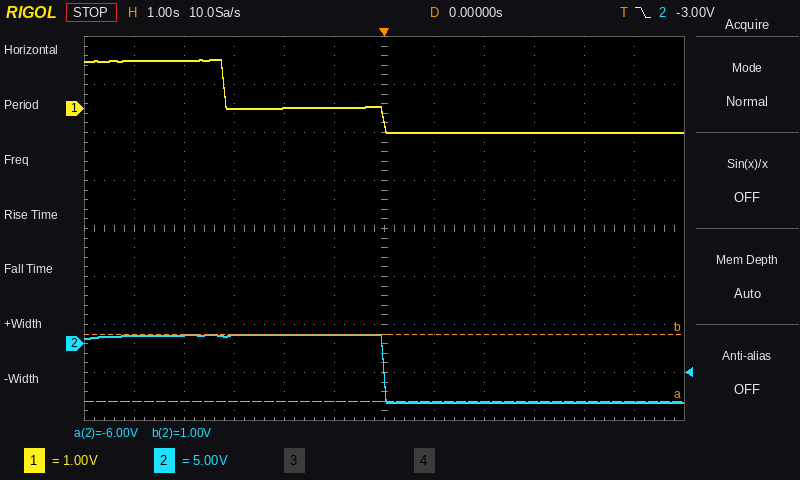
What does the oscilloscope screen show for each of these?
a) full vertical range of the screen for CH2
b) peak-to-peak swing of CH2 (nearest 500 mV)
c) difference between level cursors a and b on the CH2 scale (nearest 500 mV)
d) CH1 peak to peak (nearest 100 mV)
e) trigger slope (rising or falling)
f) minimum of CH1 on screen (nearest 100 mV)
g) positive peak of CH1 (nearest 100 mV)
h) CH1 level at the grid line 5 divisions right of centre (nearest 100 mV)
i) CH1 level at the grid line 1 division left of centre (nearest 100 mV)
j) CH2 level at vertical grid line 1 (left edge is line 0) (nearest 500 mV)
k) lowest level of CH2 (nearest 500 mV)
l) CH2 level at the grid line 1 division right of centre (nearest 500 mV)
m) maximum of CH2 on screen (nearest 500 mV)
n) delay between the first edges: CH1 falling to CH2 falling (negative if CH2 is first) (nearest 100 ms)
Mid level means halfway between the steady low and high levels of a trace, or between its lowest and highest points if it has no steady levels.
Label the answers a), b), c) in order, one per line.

a) 40 V
b) 7.0 V
c) 7.0 V
d) 1.5 V
e) falling
f) -500 mV
g) 1.0 V
h) -500 mV
i) 0.0 V
j) 1.0 V
k) -6.0 V
l) -6.0 V
m) 1.0 V
n) +3.2 s
